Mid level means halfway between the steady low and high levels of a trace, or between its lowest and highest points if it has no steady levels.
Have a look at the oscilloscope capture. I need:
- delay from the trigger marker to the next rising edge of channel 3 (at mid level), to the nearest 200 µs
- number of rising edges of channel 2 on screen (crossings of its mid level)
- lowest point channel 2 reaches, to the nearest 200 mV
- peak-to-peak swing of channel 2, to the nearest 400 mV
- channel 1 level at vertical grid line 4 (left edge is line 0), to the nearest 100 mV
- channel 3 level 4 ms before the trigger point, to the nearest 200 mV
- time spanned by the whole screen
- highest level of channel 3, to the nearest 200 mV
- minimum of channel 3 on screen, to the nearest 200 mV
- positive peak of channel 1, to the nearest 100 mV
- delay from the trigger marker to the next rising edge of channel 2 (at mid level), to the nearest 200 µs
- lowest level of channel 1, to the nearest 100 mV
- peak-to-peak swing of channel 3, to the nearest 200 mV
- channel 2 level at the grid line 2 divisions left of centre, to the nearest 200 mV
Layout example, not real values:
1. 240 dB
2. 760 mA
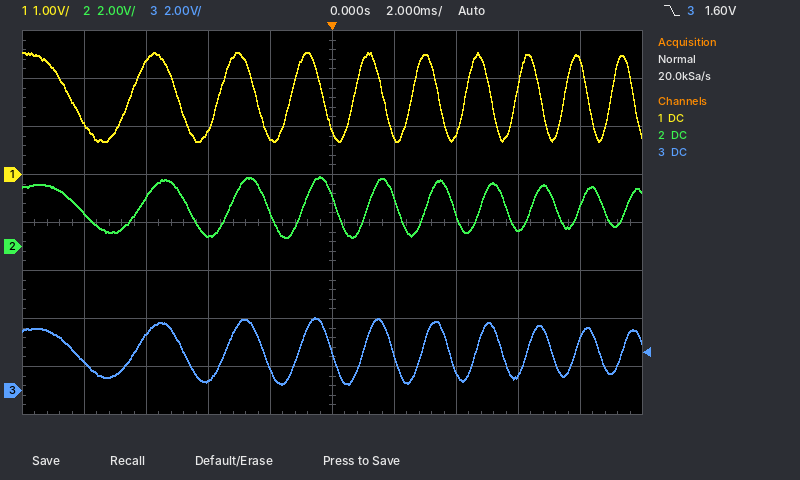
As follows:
1. 1.0 ms
2. 9
3. 400 mV
4. 2.4 V
5. 800 mV
6. 400 mV
7. 20 ms
8. 3.0 V
9. 200 mV
10. 2.5 V
11. 1.2 ms
12. 700 mV
13. 2.8 V
14. 400 mV
